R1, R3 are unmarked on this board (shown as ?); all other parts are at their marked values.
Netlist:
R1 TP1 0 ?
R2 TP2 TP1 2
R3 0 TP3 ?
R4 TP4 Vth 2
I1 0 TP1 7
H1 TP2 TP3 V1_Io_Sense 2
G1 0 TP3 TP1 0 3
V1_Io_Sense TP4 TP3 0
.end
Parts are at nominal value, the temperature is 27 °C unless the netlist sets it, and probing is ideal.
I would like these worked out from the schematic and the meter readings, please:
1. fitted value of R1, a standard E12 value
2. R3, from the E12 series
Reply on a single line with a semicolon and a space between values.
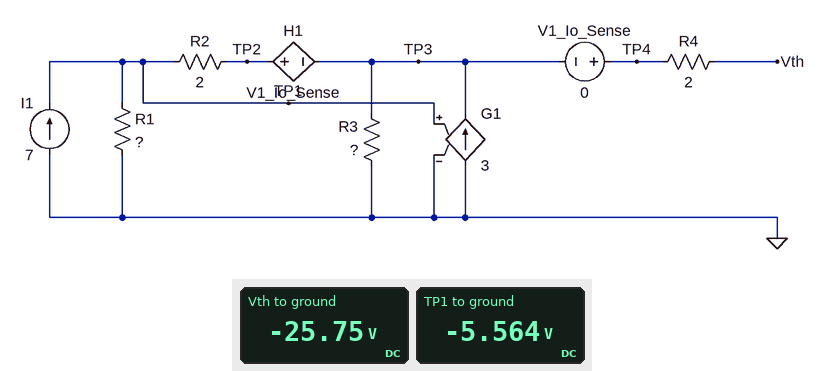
1.8 Ω; 3.9 Ω
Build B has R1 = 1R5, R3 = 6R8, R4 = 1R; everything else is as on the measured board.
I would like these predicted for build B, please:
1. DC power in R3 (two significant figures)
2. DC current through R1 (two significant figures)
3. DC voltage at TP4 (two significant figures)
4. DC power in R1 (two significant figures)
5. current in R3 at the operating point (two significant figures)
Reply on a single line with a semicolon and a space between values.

89 W; 3.0 A; -25 V; 14 W; 3.6 A
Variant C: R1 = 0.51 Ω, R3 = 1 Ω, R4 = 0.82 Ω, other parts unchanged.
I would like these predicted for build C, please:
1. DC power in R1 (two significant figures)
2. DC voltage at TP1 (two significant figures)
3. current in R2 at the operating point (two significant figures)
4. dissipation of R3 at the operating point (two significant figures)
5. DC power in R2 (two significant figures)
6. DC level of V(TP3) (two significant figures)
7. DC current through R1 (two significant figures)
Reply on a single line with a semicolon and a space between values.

57 W; 5.4 V; 3.6 A; 160 W; 26 W; 13 V; 11 A
